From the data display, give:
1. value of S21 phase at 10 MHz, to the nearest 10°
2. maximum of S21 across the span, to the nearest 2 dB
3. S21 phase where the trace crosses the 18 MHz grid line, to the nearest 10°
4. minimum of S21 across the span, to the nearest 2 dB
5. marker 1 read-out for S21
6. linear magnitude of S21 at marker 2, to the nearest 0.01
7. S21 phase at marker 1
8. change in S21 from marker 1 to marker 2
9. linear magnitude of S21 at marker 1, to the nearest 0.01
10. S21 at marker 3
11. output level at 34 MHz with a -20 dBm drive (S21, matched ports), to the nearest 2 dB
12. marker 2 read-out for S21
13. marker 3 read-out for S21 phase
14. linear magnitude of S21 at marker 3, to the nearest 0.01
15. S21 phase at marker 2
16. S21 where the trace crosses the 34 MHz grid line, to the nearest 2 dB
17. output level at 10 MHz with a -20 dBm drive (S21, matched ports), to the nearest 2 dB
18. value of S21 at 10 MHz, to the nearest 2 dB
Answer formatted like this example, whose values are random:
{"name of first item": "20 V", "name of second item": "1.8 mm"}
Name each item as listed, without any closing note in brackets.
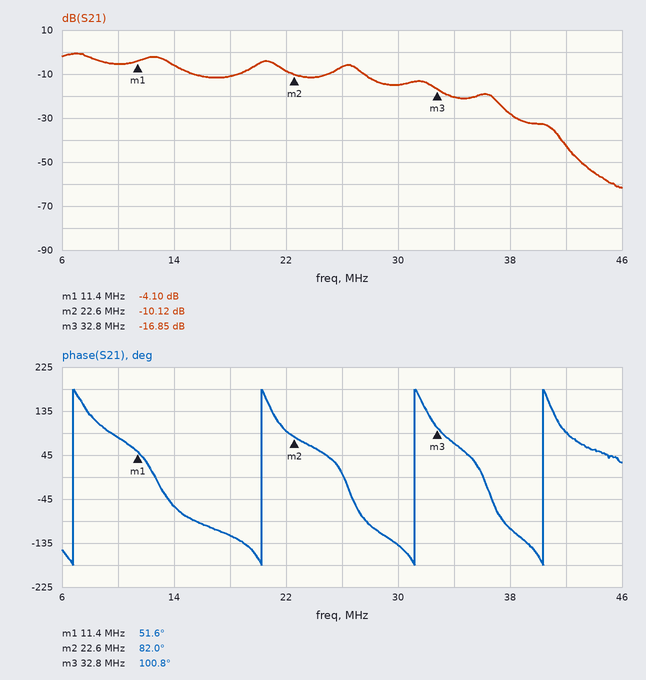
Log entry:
{"value of S21 phase at 10 MHz, to the nearest 10°": "80°", "maximum of S21 across the span, to the nearest 2 dB": "0 dB", "S21 phase where the trace crosses the 18 MHz grid line, to the nearest 10°": "-120°", "minimum of S21 across the span, to the nearest 2 dB": "-62 dB", "marker 1 read-out for S21": "-4.10 dB", "linear magnitude of S21 at marker 2, to the nearest 0.01": "0.31", "S21 phase at marker 1": "51.6°", "change in S21 from marker 1 to marker 2": "-6.02 dB", "linear magnitude of S21 at marker 1, to the nearest 0.01": "0.62", "S21 at marker 3": "-16.85 dB", "output level at 34 MHz with a -20 dBm drive (S21, matched ports), to the nearest 2 dB": "-40 dBm", "marker 2 read-out for S21": "-10.12 dB", "marker 3 read-out for S21 phase": "100.8°", "linear magnitude of S21 at marker 3, to the nearest 0.01": "0.14", "S21 phase at marker 2": "82.0°", "S21 where the trace crosses the 34 MHz grid line, to the nearest 2 dB": "-20 dB", "output level at 10 MHz with a -20 dBm drive (S21, matched ports), to the nearest 2 dB": "-26 dBm", "value of S21 at 10 MHz, to the nearest 2 dB": "-6 dB"}
